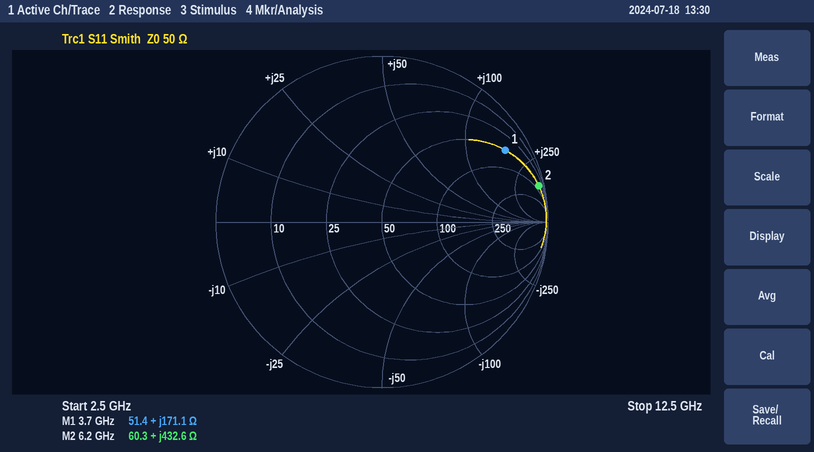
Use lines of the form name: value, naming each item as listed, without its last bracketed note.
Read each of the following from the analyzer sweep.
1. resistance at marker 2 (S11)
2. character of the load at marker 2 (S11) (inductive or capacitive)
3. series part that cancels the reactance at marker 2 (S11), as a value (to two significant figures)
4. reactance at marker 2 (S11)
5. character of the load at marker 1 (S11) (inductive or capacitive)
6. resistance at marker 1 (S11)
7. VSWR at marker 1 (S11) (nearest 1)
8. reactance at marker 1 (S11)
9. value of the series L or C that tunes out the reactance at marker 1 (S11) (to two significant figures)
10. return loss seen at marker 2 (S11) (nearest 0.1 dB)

resistance at marker 2: 60.3 Ω
character of the load at marker 2 (S11): inductive
series part that cancels the reactance at marker 2 (S11), as a value: 59 fF
reactance at marker 2: +432.6 Ω
character of the load at marker 1 (S11): inductive
resistance at marker 1: 51.4 Ω
VSWR at marker 1 (S11): 13
reactance at marker 1: +171.1 Ω
value of the series L or C that tunes out the reactance at marker 1 (S11): 250 fF
return loss seen at marker 2 (S11): 0.3 dB
